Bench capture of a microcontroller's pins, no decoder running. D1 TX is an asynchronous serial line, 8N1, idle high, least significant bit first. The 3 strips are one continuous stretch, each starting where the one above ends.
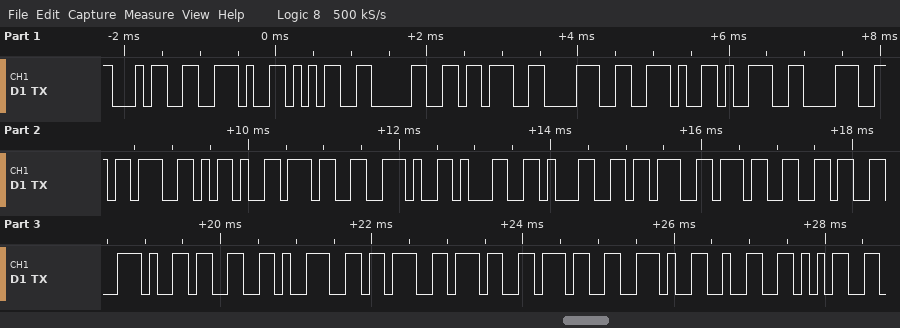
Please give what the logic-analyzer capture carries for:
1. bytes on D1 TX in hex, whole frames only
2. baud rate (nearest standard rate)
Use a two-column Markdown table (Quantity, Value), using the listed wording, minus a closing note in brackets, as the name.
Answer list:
| Quantity | Value |
|---|---|
| bytes on D1 TX in hex, whole frames only | 34 2E 35 30 3B 38 2E 39 38 3B 2D 37 2E 31 31 3B 37 36 2E 33 39 3B 37 37 2E 32 35 |
| baud rate | 9600 baud |
